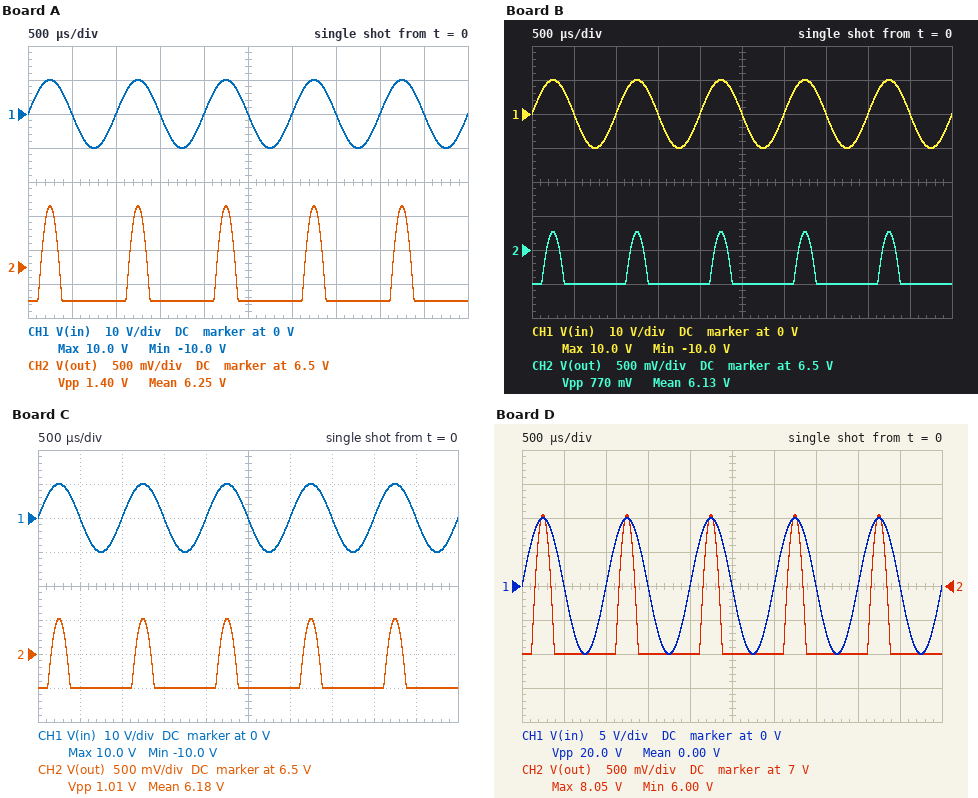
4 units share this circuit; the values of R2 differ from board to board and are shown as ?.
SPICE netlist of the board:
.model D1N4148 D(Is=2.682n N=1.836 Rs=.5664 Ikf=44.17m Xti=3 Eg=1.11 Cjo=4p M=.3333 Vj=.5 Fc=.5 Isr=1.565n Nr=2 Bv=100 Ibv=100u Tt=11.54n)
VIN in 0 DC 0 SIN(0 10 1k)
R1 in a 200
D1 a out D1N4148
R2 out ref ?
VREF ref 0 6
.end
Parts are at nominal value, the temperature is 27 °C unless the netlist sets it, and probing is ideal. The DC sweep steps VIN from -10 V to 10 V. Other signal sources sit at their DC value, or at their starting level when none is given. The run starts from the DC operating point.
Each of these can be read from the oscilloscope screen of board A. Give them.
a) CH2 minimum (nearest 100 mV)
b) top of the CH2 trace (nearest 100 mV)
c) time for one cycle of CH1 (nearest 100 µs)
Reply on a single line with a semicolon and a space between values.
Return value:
6.0 V; 7.4 V; 1.0 ms
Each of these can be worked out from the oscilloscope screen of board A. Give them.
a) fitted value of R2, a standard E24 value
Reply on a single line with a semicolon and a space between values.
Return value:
150 Ω
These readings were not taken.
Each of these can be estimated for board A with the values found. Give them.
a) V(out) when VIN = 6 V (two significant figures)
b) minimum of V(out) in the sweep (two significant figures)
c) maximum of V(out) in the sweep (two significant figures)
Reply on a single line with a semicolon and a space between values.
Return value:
6.0 V; 6.0 V; 7.4 V
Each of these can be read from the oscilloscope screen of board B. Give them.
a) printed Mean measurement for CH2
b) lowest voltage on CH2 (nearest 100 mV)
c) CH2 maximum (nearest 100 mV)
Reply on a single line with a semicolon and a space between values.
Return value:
6.13 V; 6.0 V; 6.8 V
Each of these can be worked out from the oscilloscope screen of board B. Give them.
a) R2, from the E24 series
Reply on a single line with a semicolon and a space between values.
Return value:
62 Ω
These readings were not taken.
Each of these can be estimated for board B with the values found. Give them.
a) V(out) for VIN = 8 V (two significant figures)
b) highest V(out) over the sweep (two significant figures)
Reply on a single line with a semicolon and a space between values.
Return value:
6.3 V; 6.8 V
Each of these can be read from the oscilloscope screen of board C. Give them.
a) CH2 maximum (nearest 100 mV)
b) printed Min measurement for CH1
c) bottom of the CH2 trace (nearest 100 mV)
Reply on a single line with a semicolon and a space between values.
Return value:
7.0 V; -10.0 V; 6.0 V
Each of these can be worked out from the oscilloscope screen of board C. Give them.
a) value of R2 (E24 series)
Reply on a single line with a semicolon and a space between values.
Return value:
91 Ω
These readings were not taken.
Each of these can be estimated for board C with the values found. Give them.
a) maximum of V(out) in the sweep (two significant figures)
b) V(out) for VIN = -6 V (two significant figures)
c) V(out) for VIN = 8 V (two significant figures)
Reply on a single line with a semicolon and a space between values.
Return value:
7.0 V; 6.0 V; 6.4 V
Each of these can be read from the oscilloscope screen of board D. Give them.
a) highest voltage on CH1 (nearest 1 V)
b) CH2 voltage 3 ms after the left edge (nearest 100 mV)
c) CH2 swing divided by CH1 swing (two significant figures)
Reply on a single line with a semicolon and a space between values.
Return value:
10 V; 6.0 V; 0.10
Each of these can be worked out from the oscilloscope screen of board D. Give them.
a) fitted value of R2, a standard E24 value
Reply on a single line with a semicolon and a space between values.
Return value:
330 Ω
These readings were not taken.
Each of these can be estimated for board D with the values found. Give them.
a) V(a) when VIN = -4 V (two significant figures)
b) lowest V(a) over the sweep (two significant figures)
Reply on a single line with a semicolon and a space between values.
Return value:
-4.0 V; -10 V
